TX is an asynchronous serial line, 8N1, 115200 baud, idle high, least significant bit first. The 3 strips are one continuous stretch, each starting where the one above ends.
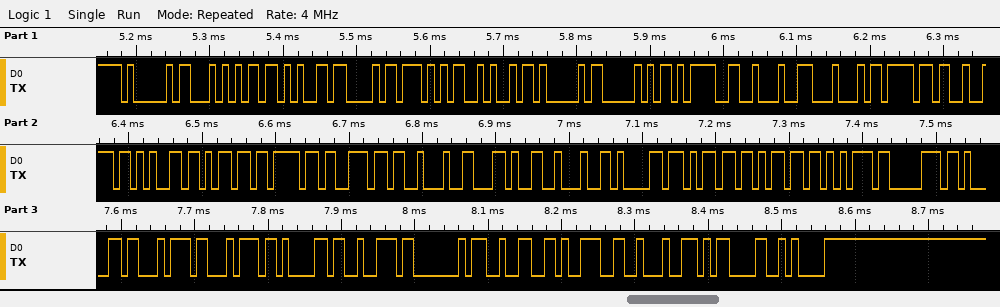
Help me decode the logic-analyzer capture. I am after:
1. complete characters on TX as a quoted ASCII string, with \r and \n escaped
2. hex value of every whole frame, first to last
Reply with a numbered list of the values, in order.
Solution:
1. "AT+CWJAP=\"Doremon\",\"ammupattar@29\"\r\n"
2. 41 54 2B 43 57 4A 41 50 3D 22 44 6F 72 65 6D 6F 6E 22 2C 22 61 6D 6D 75 70 61 74 74 61 72 40 32 39 22 0D 0A
